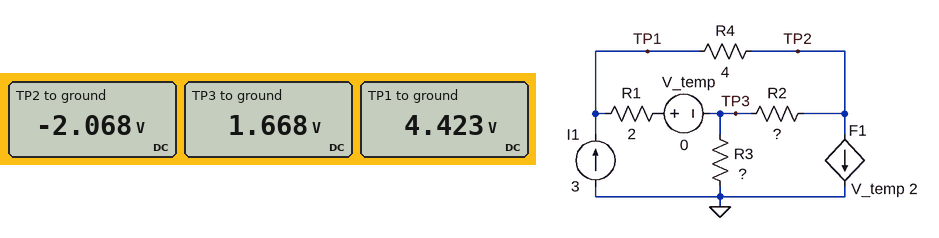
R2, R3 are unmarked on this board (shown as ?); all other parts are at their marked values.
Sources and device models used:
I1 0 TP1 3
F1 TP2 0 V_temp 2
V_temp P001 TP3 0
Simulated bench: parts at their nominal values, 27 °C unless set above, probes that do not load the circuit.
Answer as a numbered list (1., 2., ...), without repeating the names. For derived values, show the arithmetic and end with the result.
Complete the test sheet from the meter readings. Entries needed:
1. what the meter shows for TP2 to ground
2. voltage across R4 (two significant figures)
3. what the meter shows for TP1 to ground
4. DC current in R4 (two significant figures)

1. -2.068 V
2. 4.423 V - (-2.068 V) = 6.5 V
3. 4.423 V
4. (4.423 V - (-2.068 V)) / 4 Ω = 1.6 A
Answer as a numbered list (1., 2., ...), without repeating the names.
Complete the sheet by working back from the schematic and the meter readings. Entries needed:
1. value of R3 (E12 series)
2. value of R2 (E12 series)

1. 6.8 Ω
2. 3.3 Ω
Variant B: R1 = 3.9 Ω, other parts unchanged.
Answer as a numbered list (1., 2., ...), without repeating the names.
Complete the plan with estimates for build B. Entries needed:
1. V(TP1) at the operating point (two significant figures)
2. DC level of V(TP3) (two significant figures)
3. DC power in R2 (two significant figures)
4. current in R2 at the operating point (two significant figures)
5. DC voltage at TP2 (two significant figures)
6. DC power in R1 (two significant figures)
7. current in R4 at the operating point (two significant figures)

1. 8.5 V
2. 3.7 V
3. 1.6 W
4. 690 mA
5. 1.4 V
6. 5.9 W
7. 1.8 A
